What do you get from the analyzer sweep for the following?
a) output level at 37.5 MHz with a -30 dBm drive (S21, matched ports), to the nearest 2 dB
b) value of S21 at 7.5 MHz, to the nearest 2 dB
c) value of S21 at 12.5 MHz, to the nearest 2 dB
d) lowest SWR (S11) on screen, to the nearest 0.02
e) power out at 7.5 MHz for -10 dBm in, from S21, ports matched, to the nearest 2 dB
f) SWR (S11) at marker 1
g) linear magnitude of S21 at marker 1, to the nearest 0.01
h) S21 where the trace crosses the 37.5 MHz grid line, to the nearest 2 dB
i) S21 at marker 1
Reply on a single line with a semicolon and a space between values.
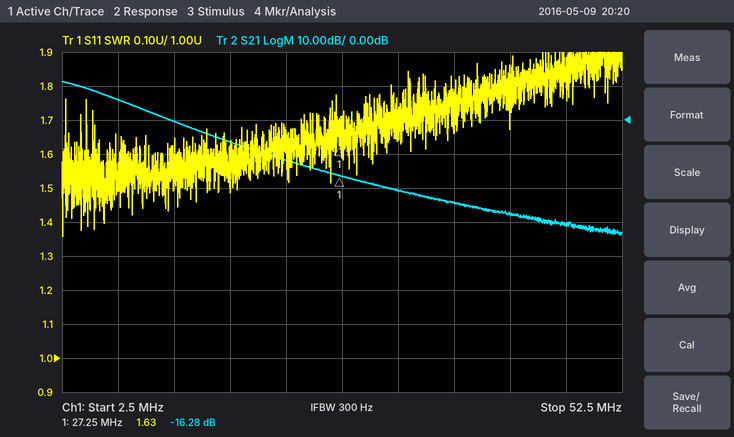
-54 dBm; 6 dB; 0 dB; 1.36; -4 dBm; 1.63; 0.15; -24 dB; -16.28 dB
